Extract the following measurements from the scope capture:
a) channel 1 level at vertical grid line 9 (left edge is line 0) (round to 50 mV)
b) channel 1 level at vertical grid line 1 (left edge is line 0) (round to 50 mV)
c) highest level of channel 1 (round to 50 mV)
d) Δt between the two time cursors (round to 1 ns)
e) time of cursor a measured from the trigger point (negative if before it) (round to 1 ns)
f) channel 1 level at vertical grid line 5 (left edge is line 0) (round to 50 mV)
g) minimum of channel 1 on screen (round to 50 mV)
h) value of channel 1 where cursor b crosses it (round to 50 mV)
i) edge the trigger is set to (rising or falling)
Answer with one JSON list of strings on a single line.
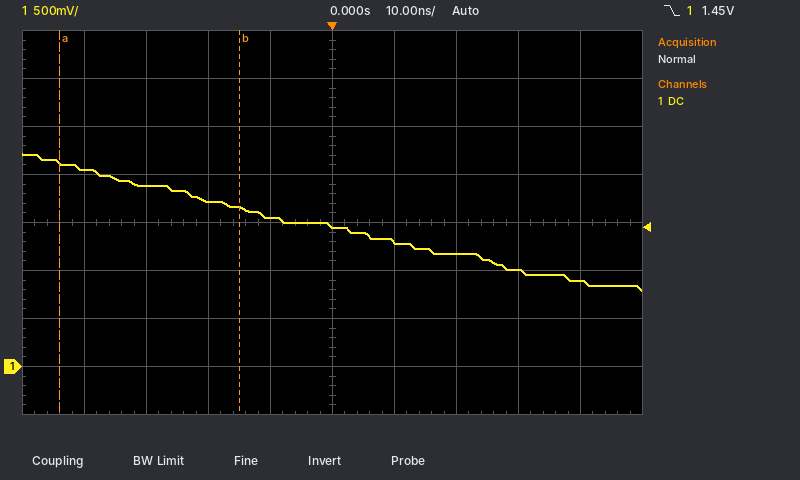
["900 mV", "2.05 V", "2.20 V", "29 ns", "-44 ns", "1.45 V", "800 mV", "1.65 V", "falling"]
